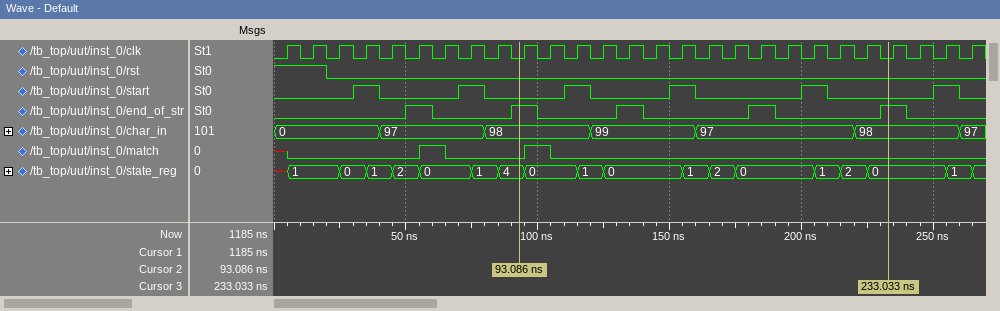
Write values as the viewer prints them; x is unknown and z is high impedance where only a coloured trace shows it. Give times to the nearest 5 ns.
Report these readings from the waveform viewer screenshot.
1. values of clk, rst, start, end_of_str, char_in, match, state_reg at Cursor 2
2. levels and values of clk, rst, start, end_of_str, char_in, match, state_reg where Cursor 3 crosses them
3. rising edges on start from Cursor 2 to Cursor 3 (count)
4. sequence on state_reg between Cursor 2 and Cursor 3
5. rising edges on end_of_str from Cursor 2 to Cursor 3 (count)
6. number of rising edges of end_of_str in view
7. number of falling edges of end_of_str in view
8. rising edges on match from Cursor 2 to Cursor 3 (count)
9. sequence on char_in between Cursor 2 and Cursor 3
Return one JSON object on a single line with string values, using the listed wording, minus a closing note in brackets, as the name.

{"values of clk, rst, start, end_of_str, char_in, match, state_reg at Cursor 2": "clk=0, rst=0, start=0, end_of_str=1, char_in=98, match=0, state_reg=4", "levels and values of clk, rst, start, end_of_str, char_in, match, state_reg where Cursor 3 crosses them": "clk=0, rst=0, start=0, end_of_str=1, char_in=98, match=0, state_reg=0", "rising edges on start from Cursor 2 to Cursor 3": "3", "sequence on state_reg between Cursor 2 and Cursor 3": "4, 0, 1, 0, 1, 2, 0, 1, 2, 0", "rising edges on end_of_str from Cursor 2 to Cursor 3": "3", "number of rising edges of end_of_str in view": "5", "number of falling edges of end_of_str in view": "5", "rising edges on match from Cursor 2 to Cursor 3": "1", "sequence on char_in between Cursor 2 and Cursor 3": "98, 99, 97, 98"}
